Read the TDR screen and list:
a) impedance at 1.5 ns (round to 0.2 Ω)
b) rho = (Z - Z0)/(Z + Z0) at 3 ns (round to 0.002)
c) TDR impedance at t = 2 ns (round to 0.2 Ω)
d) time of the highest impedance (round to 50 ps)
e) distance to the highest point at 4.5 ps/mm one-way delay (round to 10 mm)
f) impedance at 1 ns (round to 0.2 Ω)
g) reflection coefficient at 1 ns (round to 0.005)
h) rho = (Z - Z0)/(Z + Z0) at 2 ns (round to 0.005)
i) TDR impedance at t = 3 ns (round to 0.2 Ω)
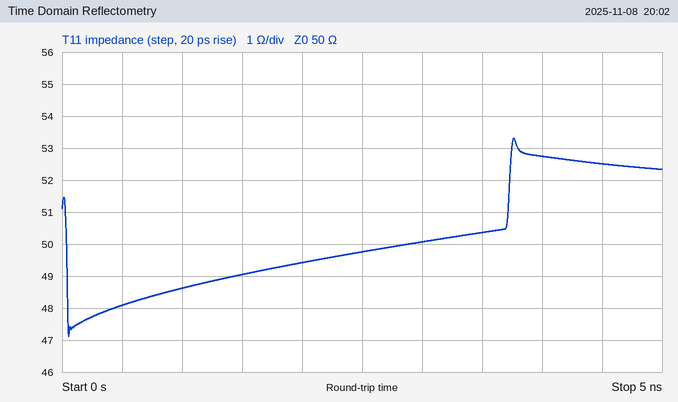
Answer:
49.0 Ω
0.000
49.4 Ω
3.75 ns
420 mm
48.6 Ω
-0.015
-0.005
50.0 Ω
